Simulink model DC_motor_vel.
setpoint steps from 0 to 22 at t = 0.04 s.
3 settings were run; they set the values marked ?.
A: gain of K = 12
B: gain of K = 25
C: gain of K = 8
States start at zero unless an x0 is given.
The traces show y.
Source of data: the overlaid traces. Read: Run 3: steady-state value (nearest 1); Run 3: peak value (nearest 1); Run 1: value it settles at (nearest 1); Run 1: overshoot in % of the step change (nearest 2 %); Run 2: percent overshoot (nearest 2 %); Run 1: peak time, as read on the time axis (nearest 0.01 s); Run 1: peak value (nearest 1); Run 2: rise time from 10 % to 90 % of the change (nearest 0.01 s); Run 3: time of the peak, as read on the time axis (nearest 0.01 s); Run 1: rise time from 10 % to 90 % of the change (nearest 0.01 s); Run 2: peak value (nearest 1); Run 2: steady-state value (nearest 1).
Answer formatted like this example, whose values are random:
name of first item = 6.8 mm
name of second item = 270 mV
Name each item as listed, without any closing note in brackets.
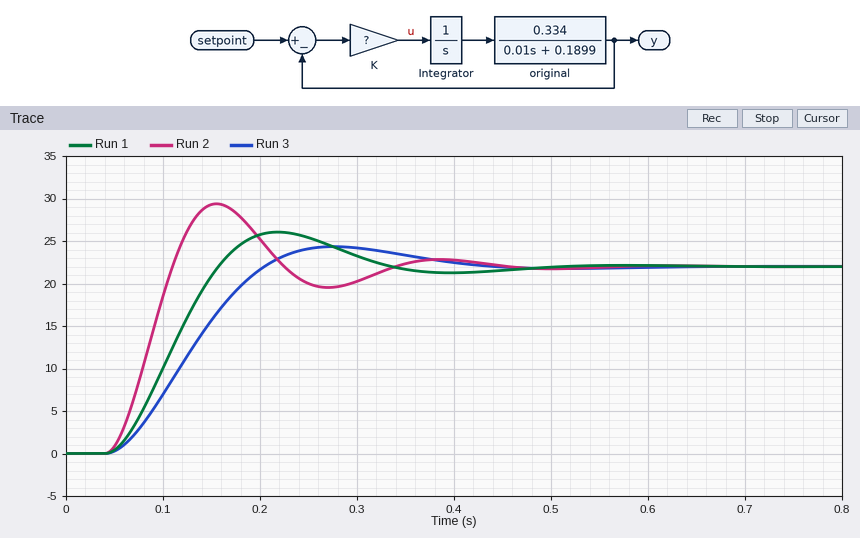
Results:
Run 3: steady-state value = 22
Run 3: peak value = 24
Run 1: value it settles at = 22
Run 1: overshoot in % of the step change = 18 %
Run 2: percent overshoot = 34 %
Run 1: peak time, as read on the time axis = 0.22 s
Run 1: peak value = 26
Run 2: rise time from 10 % to 90 % of the change = 0.05 s
Run 3: time of the peak, as read on the time axis = 0.28 s
Run 1: rise time from 10 % to 90 % of the change = 0.08 s
Run 2: peak value = 29
Run 2: steady-state value = 22
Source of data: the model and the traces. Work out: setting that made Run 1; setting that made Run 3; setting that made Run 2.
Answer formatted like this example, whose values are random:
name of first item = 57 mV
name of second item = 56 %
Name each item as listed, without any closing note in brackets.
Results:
setting that made Run 1 = A
setting that made Run 3 = C
setting that made Run 2 = B
